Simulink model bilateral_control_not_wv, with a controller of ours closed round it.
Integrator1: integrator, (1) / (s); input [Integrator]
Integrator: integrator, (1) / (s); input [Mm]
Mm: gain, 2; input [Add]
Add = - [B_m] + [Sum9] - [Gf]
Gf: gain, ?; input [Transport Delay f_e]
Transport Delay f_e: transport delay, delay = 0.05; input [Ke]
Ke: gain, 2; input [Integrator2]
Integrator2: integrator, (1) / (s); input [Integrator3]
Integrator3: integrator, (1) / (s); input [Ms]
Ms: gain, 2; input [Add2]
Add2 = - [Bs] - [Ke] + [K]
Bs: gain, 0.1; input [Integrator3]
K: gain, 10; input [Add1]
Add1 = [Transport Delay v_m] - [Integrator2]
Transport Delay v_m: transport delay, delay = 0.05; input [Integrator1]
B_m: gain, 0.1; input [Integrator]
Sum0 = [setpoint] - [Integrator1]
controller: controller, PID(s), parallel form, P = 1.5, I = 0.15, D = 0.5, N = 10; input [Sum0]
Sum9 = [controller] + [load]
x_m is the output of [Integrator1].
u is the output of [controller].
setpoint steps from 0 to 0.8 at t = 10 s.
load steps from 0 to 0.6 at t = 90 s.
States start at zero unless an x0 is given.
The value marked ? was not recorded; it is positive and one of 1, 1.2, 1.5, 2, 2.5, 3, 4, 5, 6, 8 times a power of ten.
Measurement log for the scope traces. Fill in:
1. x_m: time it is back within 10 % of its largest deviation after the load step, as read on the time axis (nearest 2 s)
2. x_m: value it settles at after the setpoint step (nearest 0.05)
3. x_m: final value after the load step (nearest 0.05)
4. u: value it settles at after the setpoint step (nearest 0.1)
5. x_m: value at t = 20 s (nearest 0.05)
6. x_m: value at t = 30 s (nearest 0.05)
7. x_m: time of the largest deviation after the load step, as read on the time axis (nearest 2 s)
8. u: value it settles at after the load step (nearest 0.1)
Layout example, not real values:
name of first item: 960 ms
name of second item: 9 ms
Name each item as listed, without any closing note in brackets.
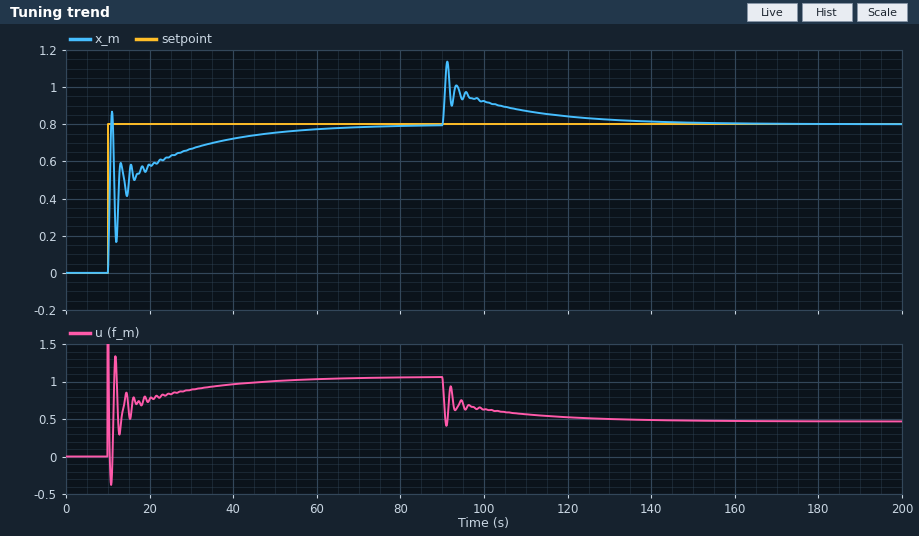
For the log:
x_m: time it is back within 10 % of its largest deviation after the load step, as read on the time axis: 124 s
x_m: value it settles at after the setpoint step: 0.80
x_m: final value after the load step: 0.80
u: value it settles at after the setpoint step: 1.1
x_m: value at t = 20 s: 0.60
x_m: value at t = 30 s: 0.65
x_m: time of the largest deviation after the load step, as read on the time axis: 92 s
u: value it settles at after the load step: 0.5
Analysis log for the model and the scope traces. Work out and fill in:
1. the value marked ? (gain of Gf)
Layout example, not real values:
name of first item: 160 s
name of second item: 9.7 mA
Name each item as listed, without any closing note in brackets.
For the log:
the value marked ?: 0.8
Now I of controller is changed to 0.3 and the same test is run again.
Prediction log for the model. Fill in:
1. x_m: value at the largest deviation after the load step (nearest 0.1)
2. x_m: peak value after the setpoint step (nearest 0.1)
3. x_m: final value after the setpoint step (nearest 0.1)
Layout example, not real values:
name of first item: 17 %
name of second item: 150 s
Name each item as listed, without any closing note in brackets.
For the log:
x_m: value at the largest deviation after the load step: 1.1
x_m: peak value after the setpoint step: 0.9
x_m: final value after the setpoint step: 0.8
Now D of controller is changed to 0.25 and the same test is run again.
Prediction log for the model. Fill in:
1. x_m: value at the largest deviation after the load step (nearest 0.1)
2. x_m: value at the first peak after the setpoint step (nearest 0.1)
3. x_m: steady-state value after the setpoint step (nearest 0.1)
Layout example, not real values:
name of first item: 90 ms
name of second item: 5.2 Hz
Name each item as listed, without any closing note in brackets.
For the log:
x_m: value at the largest deviation after the load step: 1.2
x_m: value at the first peak after the setpoint step: 0.9
x_m: steady-state value after the setpoint step: 0.8
